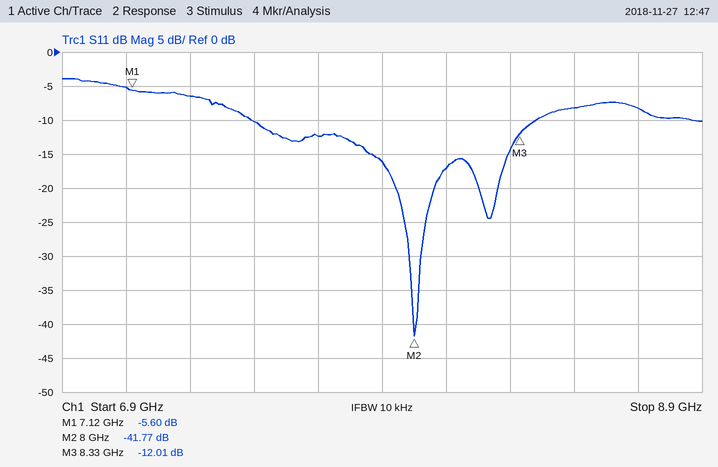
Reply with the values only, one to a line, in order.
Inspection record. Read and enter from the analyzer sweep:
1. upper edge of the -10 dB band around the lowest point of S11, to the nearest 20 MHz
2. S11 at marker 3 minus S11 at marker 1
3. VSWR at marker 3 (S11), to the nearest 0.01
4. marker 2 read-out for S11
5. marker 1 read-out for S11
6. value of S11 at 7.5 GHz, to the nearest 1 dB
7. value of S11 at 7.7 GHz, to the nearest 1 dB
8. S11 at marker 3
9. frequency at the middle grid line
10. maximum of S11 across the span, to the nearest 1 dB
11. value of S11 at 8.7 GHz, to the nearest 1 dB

8.38 GHz
-6.41 dB
1.67
-41.77 dB
-5.60 dB
-10 dB
-12 dB
-12.01 dB
7.9 GHz
-4 dB
-8 dB
